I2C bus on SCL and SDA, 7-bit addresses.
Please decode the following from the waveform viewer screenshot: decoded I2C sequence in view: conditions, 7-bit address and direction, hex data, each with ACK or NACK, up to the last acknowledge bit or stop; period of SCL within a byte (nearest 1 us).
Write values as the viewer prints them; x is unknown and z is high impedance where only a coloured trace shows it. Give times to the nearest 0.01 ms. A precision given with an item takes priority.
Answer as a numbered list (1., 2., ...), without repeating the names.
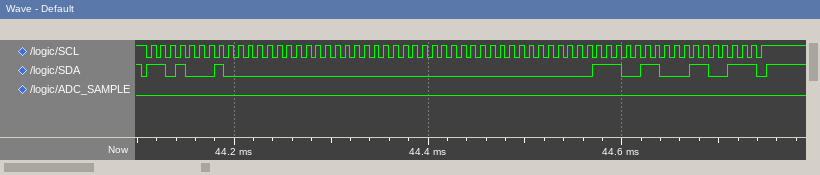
1. start, address 68 read ACK, 00 ACK, 00 ACK, 00 ACK, 00 ACK, 73 ACK, 33 NACK, stop
2. 10 us
